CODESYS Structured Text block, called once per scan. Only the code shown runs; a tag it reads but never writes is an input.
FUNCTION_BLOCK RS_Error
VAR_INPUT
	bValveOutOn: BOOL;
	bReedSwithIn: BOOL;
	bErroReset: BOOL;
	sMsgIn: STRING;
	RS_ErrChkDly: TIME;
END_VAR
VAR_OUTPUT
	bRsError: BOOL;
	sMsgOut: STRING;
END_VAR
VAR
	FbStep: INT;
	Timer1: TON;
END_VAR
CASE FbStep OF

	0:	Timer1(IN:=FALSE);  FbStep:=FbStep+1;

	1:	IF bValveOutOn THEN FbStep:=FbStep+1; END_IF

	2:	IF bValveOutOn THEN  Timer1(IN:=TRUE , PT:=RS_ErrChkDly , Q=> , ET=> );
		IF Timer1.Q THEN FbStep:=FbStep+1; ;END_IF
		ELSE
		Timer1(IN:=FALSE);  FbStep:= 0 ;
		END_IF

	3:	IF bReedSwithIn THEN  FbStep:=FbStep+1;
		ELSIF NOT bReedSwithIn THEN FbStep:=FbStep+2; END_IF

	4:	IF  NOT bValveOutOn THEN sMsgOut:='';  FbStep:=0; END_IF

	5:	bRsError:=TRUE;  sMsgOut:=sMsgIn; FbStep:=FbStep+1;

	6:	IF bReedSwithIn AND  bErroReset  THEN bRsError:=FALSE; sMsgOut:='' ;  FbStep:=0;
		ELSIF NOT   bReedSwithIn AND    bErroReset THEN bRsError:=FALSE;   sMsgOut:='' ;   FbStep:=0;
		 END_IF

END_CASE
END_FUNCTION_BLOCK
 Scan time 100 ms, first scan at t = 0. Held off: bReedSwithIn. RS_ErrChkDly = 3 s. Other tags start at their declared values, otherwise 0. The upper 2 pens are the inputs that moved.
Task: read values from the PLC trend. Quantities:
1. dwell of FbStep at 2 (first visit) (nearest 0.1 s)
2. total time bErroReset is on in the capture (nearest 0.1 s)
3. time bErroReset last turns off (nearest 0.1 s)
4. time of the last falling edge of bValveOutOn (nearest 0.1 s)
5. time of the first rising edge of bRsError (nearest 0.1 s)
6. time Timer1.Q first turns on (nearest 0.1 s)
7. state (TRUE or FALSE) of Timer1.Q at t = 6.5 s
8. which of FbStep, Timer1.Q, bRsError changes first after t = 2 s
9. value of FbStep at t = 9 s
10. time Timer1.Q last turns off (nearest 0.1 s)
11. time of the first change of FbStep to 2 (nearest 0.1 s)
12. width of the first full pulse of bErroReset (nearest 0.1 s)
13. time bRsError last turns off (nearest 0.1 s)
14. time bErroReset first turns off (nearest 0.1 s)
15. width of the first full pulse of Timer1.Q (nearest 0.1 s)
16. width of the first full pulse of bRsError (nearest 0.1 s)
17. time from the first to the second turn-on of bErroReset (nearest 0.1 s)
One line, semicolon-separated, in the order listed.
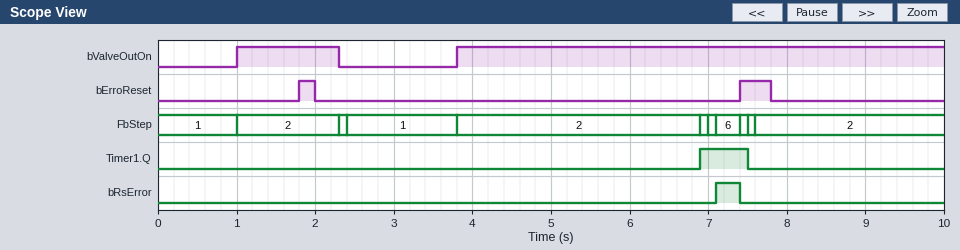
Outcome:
1.3 s; 0.6 s; 7.8 s; 2.3 s; 7.1 s; 6.9 s; FALSE; FbStep; 2; 7.5 s; 1.0 s; 0.2 s; 7.4 s; 2.0 s; 0.6 s; 0.3 s; 5.6 s
